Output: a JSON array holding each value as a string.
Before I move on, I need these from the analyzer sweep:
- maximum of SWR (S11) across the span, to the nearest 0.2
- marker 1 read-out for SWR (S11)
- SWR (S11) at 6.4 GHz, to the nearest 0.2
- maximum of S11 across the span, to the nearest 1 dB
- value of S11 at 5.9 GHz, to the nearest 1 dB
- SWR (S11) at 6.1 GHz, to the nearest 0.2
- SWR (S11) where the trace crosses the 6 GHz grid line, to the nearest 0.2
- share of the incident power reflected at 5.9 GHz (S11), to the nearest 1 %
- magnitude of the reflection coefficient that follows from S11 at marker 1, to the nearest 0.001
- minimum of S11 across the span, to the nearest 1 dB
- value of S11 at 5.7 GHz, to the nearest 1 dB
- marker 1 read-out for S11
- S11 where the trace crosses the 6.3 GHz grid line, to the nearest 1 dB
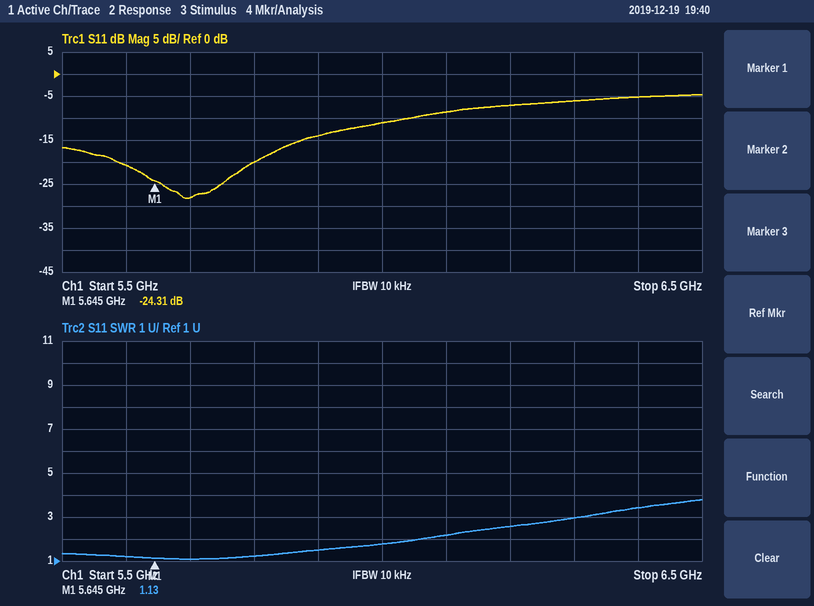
["3.8", "1.13", "3.4", "-5 dB", "-14 dB", "2.2", "1.8", "4 %", "0.061", "-28 dB", "-28 dB", "-24.31 dB", "-6 dB"]
